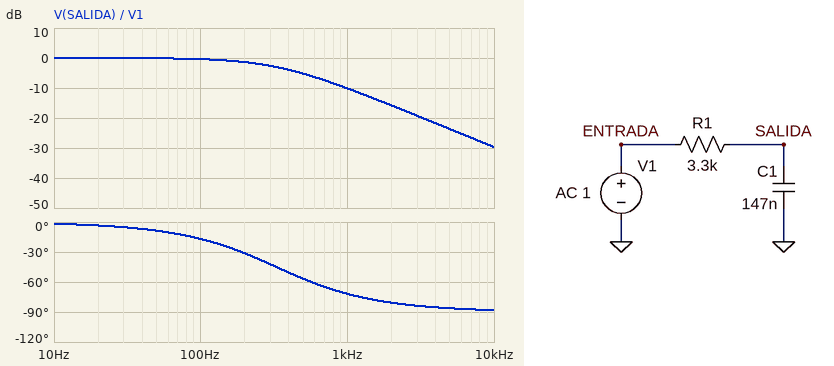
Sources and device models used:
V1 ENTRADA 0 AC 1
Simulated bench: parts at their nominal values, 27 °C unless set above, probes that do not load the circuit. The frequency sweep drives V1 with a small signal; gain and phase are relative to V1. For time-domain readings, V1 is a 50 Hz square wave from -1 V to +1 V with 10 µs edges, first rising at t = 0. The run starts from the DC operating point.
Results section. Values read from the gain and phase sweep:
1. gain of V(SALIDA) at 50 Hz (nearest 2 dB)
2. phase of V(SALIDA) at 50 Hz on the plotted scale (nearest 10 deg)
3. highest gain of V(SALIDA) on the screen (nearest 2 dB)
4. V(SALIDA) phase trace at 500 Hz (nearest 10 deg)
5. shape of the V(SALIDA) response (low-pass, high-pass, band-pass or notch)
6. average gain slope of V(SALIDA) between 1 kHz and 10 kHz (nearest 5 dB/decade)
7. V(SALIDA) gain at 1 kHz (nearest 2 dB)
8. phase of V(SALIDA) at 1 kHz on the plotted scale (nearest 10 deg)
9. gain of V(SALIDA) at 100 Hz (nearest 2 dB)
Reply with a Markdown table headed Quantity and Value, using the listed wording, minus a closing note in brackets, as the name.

| Quantity | Value |
|---|---|
| gain of V(SALIDA) at 50 Hz | 0 dB |
| phase of V(SALIDA) at 50 Hz on the plotted scale | -10 deg |
| highest gain of V(SALIDA) on the screen | 0 dB |
| V(SALIDA) phase trace at 500 Hz | -60 deg |
| shape of the V(SALIDA) response | low-pass |
| average gain slope of V(SALIDA) between 1 kHz and 10 kHz | -20 dB/decade |
| V(SALIDA) gain at 1 kHz | -10 dB |
| phase of V(SALIDA) at 1 kHz on the plotted scale | -70 deg |
| gain of V(SALIDA) at 100 Hz | 0 dB |
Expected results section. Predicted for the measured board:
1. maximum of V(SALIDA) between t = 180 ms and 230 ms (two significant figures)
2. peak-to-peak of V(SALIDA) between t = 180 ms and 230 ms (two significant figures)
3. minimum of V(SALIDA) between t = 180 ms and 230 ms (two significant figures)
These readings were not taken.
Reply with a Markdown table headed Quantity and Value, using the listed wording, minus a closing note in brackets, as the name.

| Quantity | Value |
|---|---|
| maximum of V(SALIDA) between t = 180 ms and 230 ms | 1.0 V |
| peak-to-peak of V(SALIDA) between t = 180 ms and 230 ms | 2.0 V |
| minimum of V(SALIDA) between t = 180 ms and 230 ms | -1.0 V |
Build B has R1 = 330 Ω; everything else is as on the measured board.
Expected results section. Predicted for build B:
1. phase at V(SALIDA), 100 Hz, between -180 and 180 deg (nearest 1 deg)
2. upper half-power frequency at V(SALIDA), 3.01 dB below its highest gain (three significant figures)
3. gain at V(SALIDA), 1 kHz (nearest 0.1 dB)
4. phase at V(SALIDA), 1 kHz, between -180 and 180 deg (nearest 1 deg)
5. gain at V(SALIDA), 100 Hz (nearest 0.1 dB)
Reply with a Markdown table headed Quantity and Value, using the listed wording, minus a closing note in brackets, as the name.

| Quantity | Value |
|---|---|
| phase at V(SALIDA), 100 Hz, between -180 and 180 deg | -2 deg |
| upper half-power frequency at V(SALIDA), 3.01 dB below its highest gain | 3.28 kHz |
| gain at V(SALIDA), 1 kHz | -0.4 dB |
| phase at V(SALIDA), 1 kHz, between -180 and 180 deg | -17 deg |
| gain at V(SALIDA), 100 Hz | 0 dB |
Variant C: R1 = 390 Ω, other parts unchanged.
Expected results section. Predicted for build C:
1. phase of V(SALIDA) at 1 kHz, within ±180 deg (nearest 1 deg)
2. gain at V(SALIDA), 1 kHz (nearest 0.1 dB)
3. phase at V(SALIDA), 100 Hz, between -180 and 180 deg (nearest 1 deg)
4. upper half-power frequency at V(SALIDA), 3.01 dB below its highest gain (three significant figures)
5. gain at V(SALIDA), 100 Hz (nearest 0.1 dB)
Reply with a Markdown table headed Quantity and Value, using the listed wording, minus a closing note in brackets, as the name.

| Quantity | Value |
|---|---|
| phase of V(SALIDA) at 1 kHz, within ±180 deg | -20 deg |
| gain at V(SALIDA), 1 kHz | -0.5 dB |
| phase at V(SALIDA), 100 Hz, between -180 and 180 deg | -2 deg |
| upper half-power frequency at V(SALIDA), 3.01 dB below its highest gain | 2.78 kHz |
| gain at V(SALIDA), 100 Hz | 0 dB |
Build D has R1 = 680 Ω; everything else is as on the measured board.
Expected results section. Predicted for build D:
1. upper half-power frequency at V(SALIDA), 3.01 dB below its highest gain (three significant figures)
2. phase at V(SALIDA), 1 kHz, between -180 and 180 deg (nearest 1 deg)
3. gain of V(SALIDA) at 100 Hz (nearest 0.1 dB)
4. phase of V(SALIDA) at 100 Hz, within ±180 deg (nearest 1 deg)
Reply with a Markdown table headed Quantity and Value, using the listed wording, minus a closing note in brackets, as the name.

| Quantity | Value |
|---|---|
| upper half-power frequency at V(SALIDA), 3.01 dB below its highest gain | 1.59 kHz |
| phase at V(SALIDA), 1 kHz, between -180 and 180 deg | -32 deg |
| gain of V(SALIDA) at 100 Hz | 0 dB |
| phase of V(SALIDA) at 100 Hz, within ±180 deg | -4 deg |
